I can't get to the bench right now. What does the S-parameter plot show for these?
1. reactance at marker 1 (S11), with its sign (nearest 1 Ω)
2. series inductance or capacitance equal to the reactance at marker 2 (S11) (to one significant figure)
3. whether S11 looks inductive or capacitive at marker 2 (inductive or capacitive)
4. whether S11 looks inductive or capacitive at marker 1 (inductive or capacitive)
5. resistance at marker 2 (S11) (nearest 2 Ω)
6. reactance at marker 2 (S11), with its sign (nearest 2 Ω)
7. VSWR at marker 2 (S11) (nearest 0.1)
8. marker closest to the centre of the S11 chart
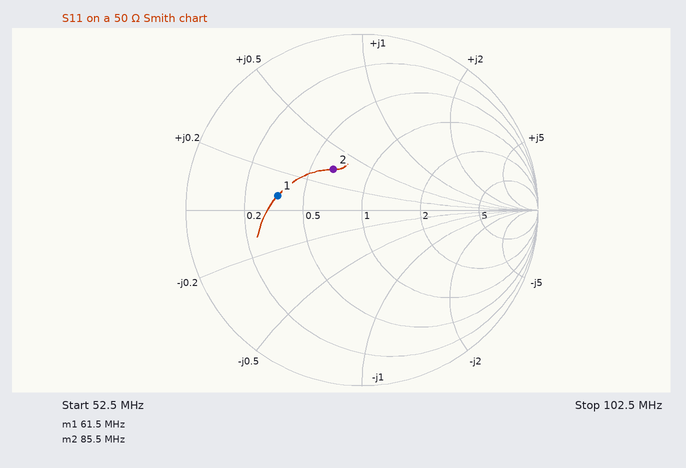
+4 Ω
30 nH
inductive
inductive
32 Ω
+16 Ω
1.8
marker 2
